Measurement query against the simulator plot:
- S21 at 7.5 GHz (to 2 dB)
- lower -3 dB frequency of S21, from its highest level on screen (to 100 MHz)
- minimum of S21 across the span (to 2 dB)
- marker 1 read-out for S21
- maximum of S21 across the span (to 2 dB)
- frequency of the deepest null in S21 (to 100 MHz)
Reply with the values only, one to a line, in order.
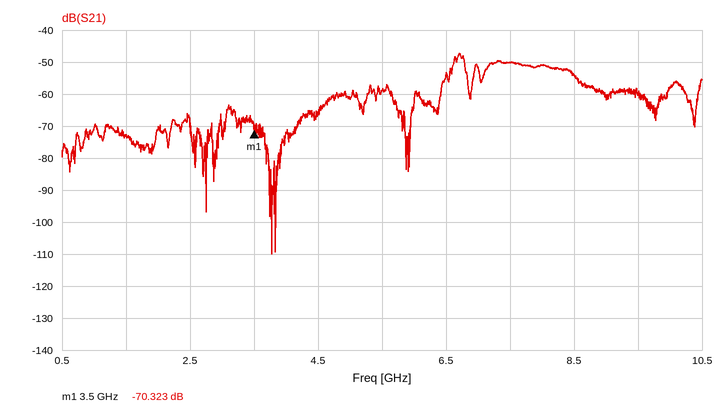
-50 dB
6.6 GHz
-110 dB
-70.323 dB
-48 dB
3.8 GHz
